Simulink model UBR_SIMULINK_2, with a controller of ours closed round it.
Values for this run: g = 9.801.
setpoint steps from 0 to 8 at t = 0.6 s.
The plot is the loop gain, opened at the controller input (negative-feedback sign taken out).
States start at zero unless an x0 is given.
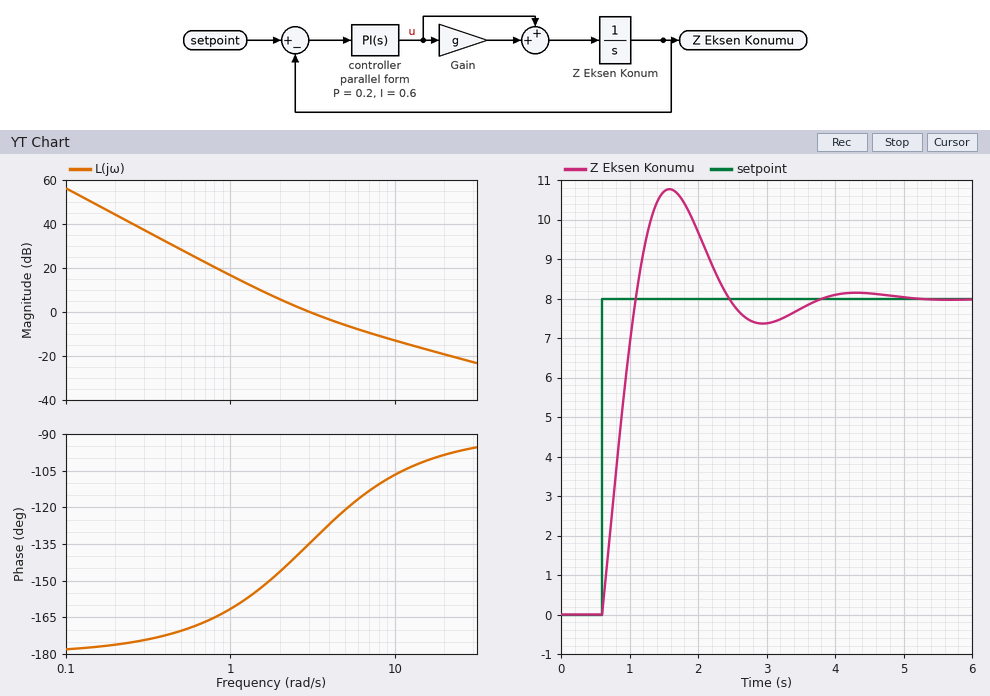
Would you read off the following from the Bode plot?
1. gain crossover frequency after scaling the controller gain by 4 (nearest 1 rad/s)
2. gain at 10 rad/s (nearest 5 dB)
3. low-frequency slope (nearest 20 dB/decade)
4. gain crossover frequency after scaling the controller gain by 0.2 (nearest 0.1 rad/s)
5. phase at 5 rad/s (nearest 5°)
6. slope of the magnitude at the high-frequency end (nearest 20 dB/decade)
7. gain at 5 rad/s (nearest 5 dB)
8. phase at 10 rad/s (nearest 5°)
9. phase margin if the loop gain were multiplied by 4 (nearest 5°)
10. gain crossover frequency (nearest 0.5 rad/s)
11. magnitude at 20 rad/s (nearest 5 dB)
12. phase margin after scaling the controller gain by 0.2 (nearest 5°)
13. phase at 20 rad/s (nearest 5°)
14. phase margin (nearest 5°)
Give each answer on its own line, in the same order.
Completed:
9 rad/s
-15 dB
-40 dB/decade
1.2 rad/s
-120°
-20 dB/decade
-5 dB
-105°
70°
3.0 rad/s
-20 dB
20°
-100°
45°
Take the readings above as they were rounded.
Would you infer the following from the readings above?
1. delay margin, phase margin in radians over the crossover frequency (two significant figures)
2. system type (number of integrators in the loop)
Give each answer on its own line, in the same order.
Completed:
0.26 s
2
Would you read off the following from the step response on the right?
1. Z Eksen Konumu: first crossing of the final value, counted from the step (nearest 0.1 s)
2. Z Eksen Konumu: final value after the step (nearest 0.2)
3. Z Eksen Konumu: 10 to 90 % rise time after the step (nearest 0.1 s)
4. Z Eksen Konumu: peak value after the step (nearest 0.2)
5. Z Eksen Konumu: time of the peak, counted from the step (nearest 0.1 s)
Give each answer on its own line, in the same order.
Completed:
0.5 s
8.0
0.4 s
10.8
1.0 s
